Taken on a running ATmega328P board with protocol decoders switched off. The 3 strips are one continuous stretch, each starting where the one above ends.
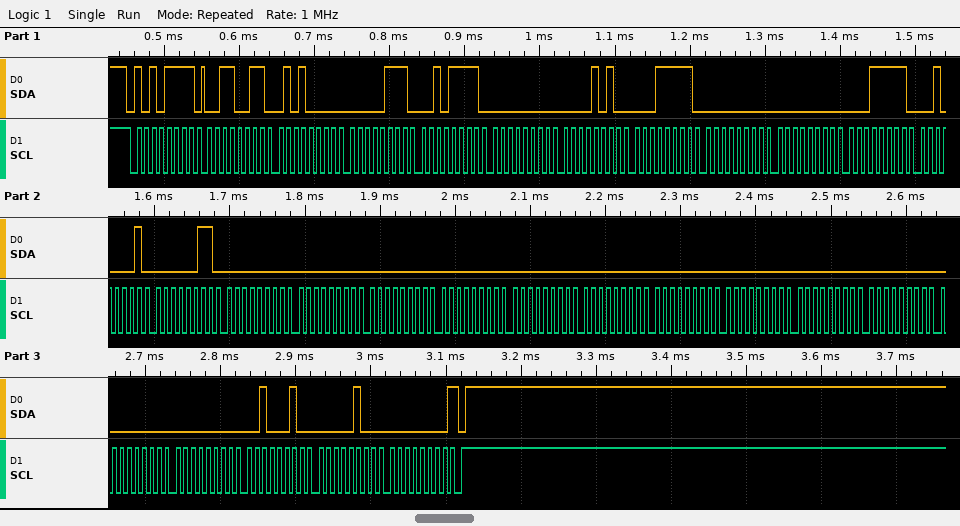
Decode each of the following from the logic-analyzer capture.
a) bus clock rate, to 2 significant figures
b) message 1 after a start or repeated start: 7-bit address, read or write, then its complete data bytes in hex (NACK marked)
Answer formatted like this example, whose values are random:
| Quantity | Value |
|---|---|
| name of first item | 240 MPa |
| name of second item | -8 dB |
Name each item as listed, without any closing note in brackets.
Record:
| Quantity | Value |
|---|---|
| bus clock rate, to 2 significant figures | 100 kHz |
| message 1 after a start or repeated start: 7-bit address, read or write, then its complete data bytes in hex | 0x57 read: 33 50 07 2F 00 0A 1F 00 00 1F 21 03 00 00 00 00 00 00 00 00 00 00 00 00 22 04 00 NACK |
